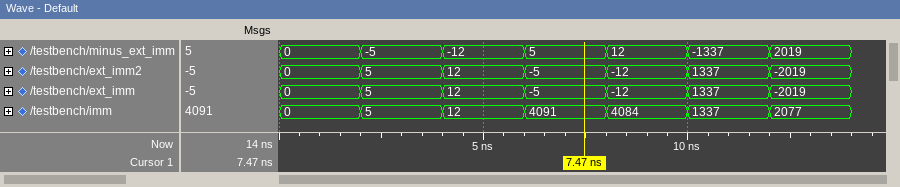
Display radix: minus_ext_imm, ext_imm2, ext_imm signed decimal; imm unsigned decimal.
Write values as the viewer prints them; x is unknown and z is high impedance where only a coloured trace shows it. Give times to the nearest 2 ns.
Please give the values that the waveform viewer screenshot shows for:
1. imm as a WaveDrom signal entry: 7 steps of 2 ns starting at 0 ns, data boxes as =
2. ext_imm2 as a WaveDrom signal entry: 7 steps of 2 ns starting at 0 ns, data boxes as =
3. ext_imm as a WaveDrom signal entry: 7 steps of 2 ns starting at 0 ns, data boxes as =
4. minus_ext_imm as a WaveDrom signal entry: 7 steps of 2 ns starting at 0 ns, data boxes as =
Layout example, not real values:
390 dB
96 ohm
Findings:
{name: 'imm', wave: '=======', data: '0 5 12 4091 4084 1337 2077'}
{name: 'ext_imm2', wave: '=======', data: '0 5 12 -5 -12 1337 -2019'}
{name: 'ext_imm', wave: '=======', data: '0 5 12 -5 -12 1337 -2019'}
{name: 'minus_ext_imm', wave: '=======', data: '0 -5 -12 5 12 -1337 2019'}
